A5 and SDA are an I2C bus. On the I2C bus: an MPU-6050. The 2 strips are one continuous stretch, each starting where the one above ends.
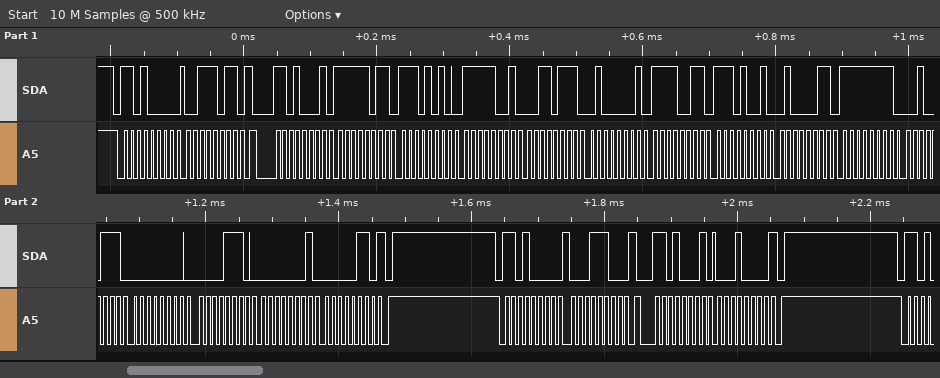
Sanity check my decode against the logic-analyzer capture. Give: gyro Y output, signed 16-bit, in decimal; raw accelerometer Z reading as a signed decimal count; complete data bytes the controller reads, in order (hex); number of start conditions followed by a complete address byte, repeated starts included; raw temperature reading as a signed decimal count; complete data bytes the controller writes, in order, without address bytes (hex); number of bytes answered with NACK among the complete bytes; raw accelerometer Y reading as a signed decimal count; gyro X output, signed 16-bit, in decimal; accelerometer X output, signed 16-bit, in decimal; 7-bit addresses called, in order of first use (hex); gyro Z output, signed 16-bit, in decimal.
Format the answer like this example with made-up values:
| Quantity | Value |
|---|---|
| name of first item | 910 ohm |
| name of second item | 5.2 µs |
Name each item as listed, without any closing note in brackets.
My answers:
| Quantity | Value |
|---|---|
| gyro Y output, signed 16-bit, in decimal | 14 |
| raw accelerometer Z reading as a signed decimal count | 16883 |
| complete data bytes the controller reads, in order | FB EA F9 37 41 F3 E9 43 FF 27 00 0E 01 06 10 |
| number of start conditions followed by a complete address byte, repeated starts included | 4 |
| raw temperature reading as a signed decimal count | -5821 |
| complete data bytes the controller writes, in order, without address bytes | 3B 1C |
| number of bytes answered with NACK among the complete bytes | 2 |
| raw accelerometer Y reading as a signed decimal count | -1737 |
| gyro X output, signed 16-bit, in decimal | -217 |
| accelerometer X output, signed 16-bit, in decimal | -1046 |
| 7-bit addresses called, in order of first use | 0x68 |
| gyro Z output, signed 16-bit, in decimal | 262 |
